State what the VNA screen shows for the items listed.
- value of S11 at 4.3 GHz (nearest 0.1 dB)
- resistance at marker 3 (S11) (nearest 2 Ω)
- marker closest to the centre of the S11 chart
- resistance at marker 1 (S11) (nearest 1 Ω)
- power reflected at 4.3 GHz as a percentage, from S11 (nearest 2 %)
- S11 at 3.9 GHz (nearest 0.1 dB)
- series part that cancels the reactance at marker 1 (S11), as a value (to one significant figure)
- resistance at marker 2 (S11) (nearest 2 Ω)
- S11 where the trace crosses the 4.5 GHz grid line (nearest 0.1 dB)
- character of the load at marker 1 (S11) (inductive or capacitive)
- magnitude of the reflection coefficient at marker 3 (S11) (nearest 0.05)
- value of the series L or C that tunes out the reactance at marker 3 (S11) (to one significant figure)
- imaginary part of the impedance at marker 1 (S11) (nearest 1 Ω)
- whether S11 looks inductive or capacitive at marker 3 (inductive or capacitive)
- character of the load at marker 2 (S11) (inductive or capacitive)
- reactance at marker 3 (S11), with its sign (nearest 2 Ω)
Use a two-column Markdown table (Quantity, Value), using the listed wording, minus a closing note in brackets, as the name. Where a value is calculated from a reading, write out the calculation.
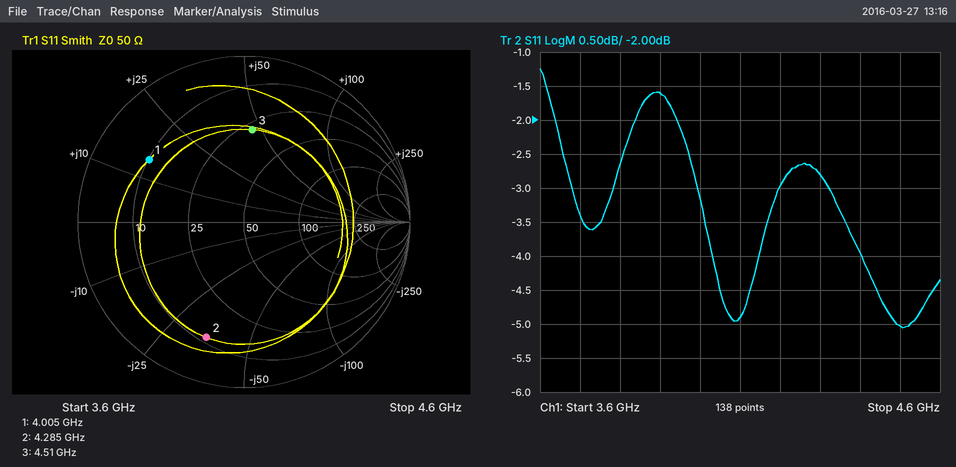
| Quantity | Value |
|---|---|
| value of S11 at 4.3 GHz | -2.8 dB |
| resistance at marker 3 (S11) | 28 Ω |
| marker closest to the centre of the S11 chart | marker 3 |
| resistance at marker 1 (S11) | 10 Ω |
| power reflected at 4.3 GHz as a percentage, from S11 | 10^(-2.8/10) ≈ 52 % |
| S11 at 3.9 GHz | -1.6 dB |
| series part that cancels the reactance at marker 1 (S11), as a value | C = 1/(2π × 4.005 GHz × 14 Ω) ≈ 3 pF |
| resistance at marker 2 (S11) | 12 Ω |
| S11 where the trace crosses the 4.5 GHz grid line | -5.0 dB |
| character of the load at marker 1 (S11) | inductive |
| magnitude of the reflection coefficient at marker 3 (S11) | 0.55 |
| value of the series L or C that tunes out the reactance at marker 3 (S11) | C = 1/(2π × 4.51 GHz × 46 Ω) ≈ 767 fF, so 800 fF to one significant figure |
| imaginary part of the impedance at marker 1 (S11) | +14 Ω |
| whether S11 looks inductive or capacitive at marker 3 | inductive |
| character of the load at marker 2 (S11) | capacitive |
| reactance at marker 3 (S11), with its sign | +46 Ω |
